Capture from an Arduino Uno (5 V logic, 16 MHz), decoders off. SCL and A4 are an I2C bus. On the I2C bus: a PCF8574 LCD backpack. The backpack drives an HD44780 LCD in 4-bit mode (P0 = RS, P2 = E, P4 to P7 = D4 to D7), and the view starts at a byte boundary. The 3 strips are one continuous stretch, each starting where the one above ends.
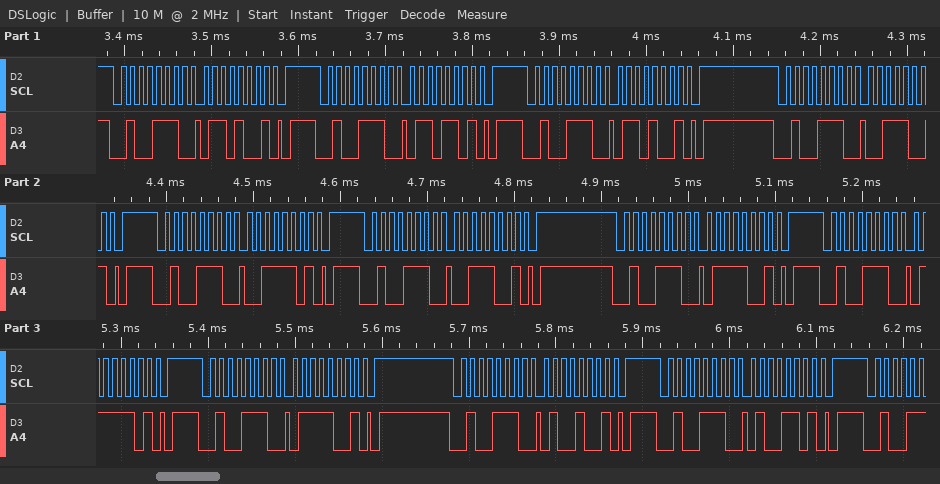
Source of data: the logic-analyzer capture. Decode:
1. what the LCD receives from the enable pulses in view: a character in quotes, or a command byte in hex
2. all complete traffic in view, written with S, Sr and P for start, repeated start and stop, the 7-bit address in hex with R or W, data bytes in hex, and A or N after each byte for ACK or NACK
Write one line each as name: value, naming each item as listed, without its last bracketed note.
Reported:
what the LCD receives from the enable pulses in view: a character in quotes, or a command byte in hex: 'c'
all complete traffic in view, written with S, Sr and P for start, repeated start and stop, the 7-bit address in hex with R or W, data bytes in hex, and A or N after each byte for ACK or NACK: S 27W A 69 A P S 27W A 6D A P S 27W A 69 A P S 27W A 39 A P S 27W A 3D A P S 27W A 39 A P S 27W A 79 A P S 27W A 7D A P S 27W A 79 A P S 27W A 49 A P S 27W A 4D A P
